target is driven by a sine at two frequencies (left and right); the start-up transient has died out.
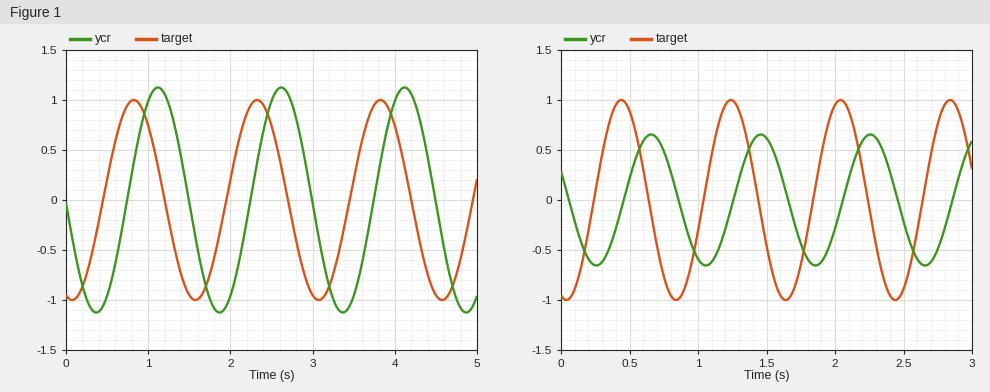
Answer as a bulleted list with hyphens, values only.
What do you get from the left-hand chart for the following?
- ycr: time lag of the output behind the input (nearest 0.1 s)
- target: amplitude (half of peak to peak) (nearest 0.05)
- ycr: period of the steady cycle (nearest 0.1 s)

- 0.3 s
- 1.00
- 1.5 s
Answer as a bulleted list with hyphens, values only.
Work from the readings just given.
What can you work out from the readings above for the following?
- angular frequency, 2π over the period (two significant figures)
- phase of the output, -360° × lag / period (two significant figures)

- 4.2 rad/s
- -72°
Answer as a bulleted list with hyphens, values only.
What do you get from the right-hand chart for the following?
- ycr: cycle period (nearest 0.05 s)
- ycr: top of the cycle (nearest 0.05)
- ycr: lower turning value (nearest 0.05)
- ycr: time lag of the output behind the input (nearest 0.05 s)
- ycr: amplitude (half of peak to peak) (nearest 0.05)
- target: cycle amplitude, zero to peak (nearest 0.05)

- 0.80 s
- 0.65
- -0.65
- 0.20 s
- 0.65
- 1.00
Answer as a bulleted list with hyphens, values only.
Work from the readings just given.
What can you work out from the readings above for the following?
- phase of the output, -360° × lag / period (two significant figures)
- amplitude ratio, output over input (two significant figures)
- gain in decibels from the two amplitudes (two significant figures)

- -90°
- 0.65
- -3.7 dB
